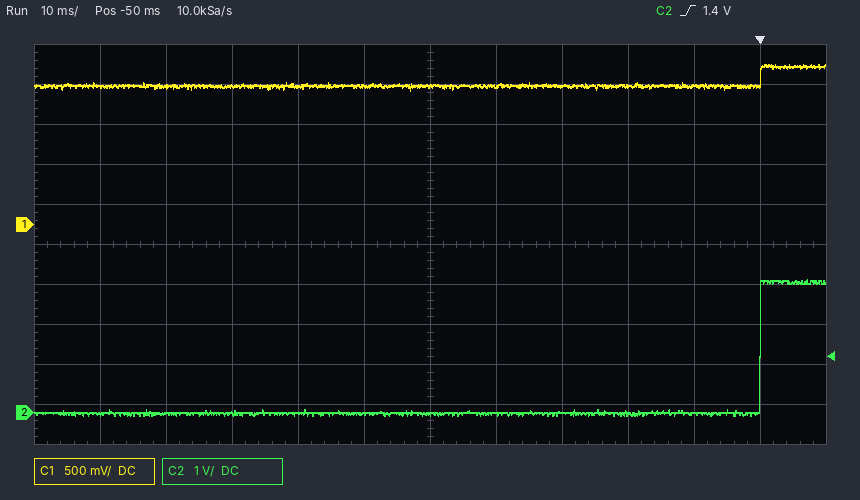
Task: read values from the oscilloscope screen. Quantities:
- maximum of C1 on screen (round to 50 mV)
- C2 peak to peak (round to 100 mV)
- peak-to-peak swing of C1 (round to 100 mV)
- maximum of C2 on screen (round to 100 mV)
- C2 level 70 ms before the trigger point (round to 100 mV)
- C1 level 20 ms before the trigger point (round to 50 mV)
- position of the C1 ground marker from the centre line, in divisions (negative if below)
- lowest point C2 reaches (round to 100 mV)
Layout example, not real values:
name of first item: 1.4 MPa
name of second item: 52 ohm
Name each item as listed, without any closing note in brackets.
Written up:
maximum of C1 on screen: 2.00 V
C2 peak to peak: 3.4 V
peak-to-peak swing of C1: 300 mV
maximum of C2 on screen: 3.3 V
C2 level 70 ms before the trigger point: 0.0 V
C1 level 20 ms before the trigger point: 1.75 V
position of the C1 ground marker from the centre line, in divisions: +0.5 div
lowest point C2 reaches: -100 mV
